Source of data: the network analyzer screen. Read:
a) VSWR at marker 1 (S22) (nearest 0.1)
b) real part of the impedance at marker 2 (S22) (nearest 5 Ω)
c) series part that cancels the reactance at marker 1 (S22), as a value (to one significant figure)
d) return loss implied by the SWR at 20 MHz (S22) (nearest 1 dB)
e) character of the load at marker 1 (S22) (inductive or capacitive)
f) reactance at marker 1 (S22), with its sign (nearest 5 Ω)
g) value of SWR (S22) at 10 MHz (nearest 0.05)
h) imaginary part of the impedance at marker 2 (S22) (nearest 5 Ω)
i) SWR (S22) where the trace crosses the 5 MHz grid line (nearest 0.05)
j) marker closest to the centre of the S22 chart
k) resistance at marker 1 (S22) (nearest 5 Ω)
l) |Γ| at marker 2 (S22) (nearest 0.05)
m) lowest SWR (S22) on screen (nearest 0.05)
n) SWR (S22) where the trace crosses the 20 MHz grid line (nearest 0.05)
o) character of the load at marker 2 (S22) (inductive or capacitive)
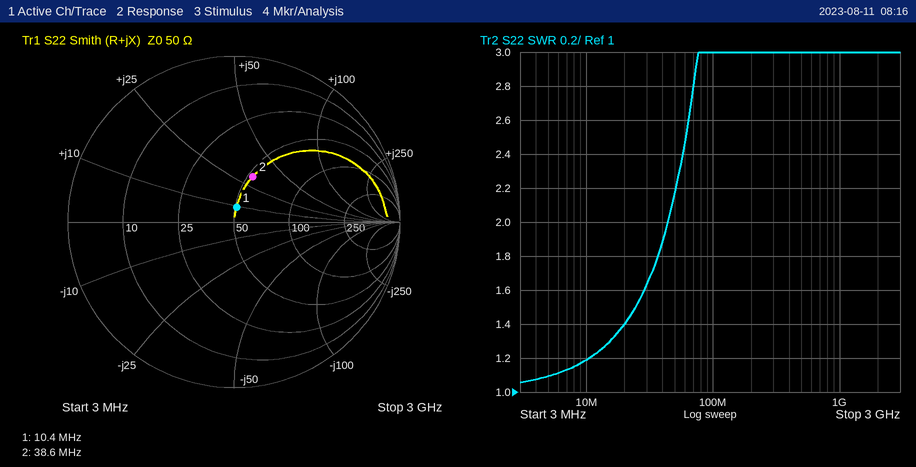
1.2
55 Ω
2 nF
16 dB
inductive
+10 Ω
1.20
+30 Ω
1.10
marker 1
50 Ω
0.30
1.05
1.40
inductive
